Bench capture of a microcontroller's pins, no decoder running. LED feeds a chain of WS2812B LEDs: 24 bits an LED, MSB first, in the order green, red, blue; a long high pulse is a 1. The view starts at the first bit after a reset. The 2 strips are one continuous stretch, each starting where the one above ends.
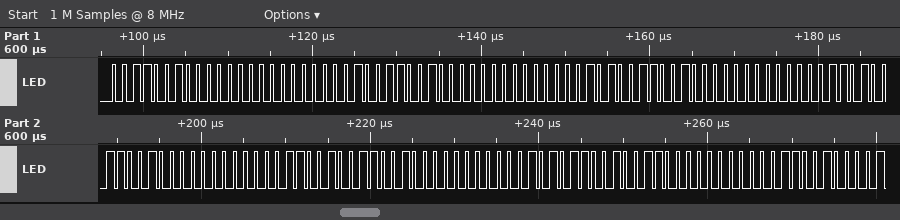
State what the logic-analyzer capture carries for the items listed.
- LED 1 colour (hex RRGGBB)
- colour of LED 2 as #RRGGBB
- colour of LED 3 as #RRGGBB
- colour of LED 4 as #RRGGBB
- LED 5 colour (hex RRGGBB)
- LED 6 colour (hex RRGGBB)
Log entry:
#003201
#003205
#00320D
#003219
#00322B
#002632
